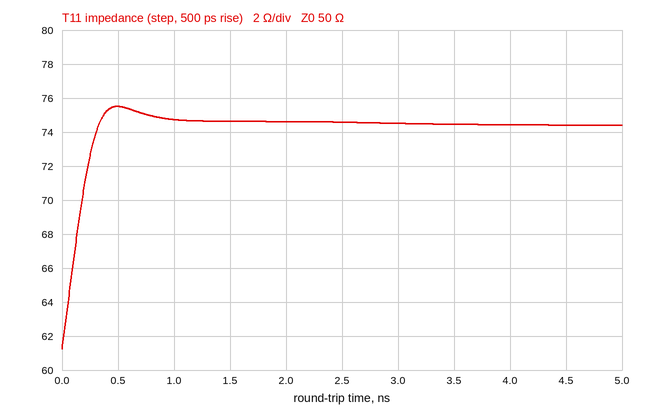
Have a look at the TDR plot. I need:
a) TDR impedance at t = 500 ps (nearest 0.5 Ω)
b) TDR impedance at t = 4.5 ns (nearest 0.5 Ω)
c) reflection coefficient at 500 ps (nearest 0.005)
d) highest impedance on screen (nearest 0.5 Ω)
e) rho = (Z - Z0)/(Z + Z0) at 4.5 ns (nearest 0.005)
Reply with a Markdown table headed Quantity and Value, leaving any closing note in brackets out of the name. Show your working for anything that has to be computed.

| Quantity | Value |
|---|---|
| TDR impedance at t = 500 ps | 75.5 Ω |
| TDR impedance at t = 4.5 ns | 74.5 Ω |
| reflection coefficient at 500 ps | (75.5 − 50)/(75.5 + 50) ≈ +0.203, so +0.205 to the nearest 0.005 |
| highest impedance on screen | 75.5 Ω |
| rho = (Z - Z0)/(Z + Z0) at 4.5 ns | (74.5 − 50)/(74.5 + 50) ≈ +0.197, so +0.195 to the nearest 0.005 |
